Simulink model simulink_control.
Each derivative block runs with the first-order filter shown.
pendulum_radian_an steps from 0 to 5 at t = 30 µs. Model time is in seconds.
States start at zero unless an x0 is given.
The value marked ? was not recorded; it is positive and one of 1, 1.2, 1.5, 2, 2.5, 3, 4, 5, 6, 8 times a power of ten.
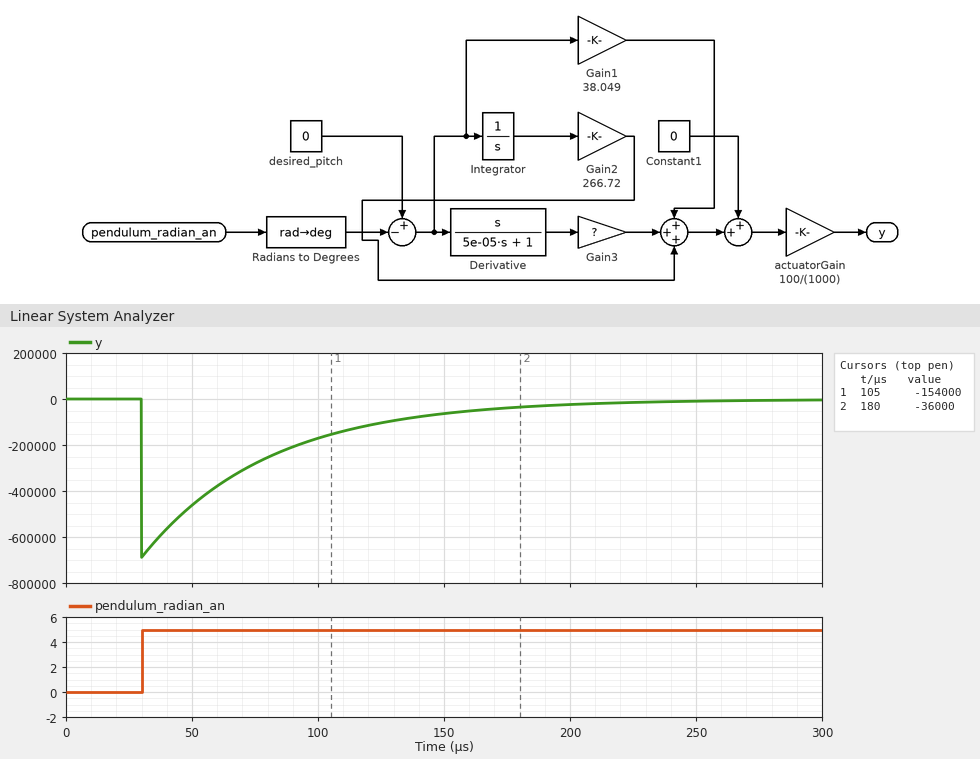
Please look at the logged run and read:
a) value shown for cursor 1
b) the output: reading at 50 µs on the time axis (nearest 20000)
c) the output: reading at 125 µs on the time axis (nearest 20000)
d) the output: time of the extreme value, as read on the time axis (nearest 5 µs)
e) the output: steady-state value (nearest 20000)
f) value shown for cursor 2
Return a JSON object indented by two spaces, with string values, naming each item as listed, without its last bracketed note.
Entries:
{
  "value shown for cursor 1": "-154000",
  "the output: reading at 50 µs on the time axis": "-460000",
  "the output: reading at 125 µs on the time axis": "-100000",
  "the output: time of the extreme value, as read on the time axis": "30 µs",
  "the output: steady-state value": "0",
  "value shown for cursor 2": "-36000"
}
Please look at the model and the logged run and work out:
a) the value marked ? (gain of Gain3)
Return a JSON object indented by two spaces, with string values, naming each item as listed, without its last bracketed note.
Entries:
{
  "the value marked ?": "1.2"
}
